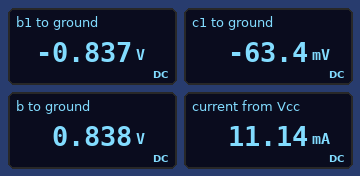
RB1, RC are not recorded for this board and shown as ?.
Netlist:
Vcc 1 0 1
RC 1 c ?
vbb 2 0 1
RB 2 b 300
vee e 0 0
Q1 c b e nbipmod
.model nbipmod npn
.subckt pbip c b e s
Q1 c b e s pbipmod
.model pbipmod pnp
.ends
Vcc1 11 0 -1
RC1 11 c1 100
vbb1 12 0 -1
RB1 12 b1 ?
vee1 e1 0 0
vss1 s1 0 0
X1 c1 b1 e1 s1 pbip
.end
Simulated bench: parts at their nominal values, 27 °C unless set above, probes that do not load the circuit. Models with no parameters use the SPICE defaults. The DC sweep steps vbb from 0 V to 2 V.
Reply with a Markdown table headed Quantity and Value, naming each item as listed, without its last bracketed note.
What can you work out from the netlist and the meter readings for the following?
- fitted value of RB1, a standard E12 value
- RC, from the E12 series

| Quantity | Value |
|---|---|
| fitted value of RB1, a standard E12 value | 150 Ω |
| RC, from the E12 series | 82 Ω |
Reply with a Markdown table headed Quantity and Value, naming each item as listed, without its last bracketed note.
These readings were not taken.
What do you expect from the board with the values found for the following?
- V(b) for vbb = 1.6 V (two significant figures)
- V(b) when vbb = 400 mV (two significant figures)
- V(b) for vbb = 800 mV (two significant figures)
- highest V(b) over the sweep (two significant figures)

| Quantity | Value |
|---|---|
| V(b) for vbb = 1.6 V | 850 mV |
| V(b) when vbb = 400 mV | 400 mV |
| V(b) for vbb = 800 mV | 790 mV |
| highest V(b) over the sweep | 850 mV |
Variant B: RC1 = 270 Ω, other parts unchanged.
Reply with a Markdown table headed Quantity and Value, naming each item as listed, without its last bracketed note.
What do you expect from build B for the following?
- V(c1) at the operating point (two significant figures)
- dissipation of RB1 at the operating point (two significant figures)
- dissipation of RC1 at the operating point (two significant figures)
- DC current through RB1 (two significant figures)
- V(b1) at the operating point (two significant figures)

| Quantity | Value |
|---|---|
| V(c1) at the operating point | -42 mV |
| dissipation of RB1 at the operating point | 220 µW |
| dissipation of RC1 at the operating point | 3.4 mW |
| DC current through RB1 | 1.2 mA |
| V(b1) at the operating point | -820 mV |
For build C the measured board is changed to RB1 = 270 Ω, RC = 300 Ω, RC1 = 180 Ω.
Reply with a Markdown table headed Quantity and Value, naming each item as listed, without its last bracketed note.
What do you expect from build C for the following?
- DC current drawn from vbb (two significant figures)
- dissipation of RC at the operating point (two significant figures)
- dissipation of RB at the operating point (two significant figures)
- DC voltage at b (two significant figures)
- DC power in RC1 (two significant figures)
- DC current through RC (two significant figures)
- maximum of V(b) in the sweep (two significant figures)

| Quantity | Value |
|---|---|
| DC current drawn from vbb | 630 µA |
| dissipation of RC at the operating point | 3.0 mW |
| dissipation of RB at the operating point | 120 µW |
| DC voltage at b | 810 mV |
| DC power in RC1 | 4.9 mW |
| DC current through RC | 3.2 mA |
| maximum of V(b) in the sweep | 840 mV |
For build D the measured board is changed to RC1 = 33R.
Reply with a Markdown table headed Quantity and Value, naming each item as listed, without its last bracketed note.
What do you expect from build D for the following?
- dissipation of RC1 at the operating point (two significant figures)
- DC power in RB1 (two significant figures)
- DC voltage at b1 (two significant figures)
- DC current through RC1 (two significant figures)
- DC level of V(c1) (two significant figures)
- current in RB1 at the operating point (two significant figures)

| Quantity | Value |
|---|---|
| dissipation of RC1 at the operating point | 25 mW |
| DC power in RB1 | 130 µW |
| DC voltage at b1 | -860 mV |
| DC current through RC1 | 27 mA |
| DC level of V(c1) | -98 mV |
| current in RB1 at the operating point | 930 µA |
